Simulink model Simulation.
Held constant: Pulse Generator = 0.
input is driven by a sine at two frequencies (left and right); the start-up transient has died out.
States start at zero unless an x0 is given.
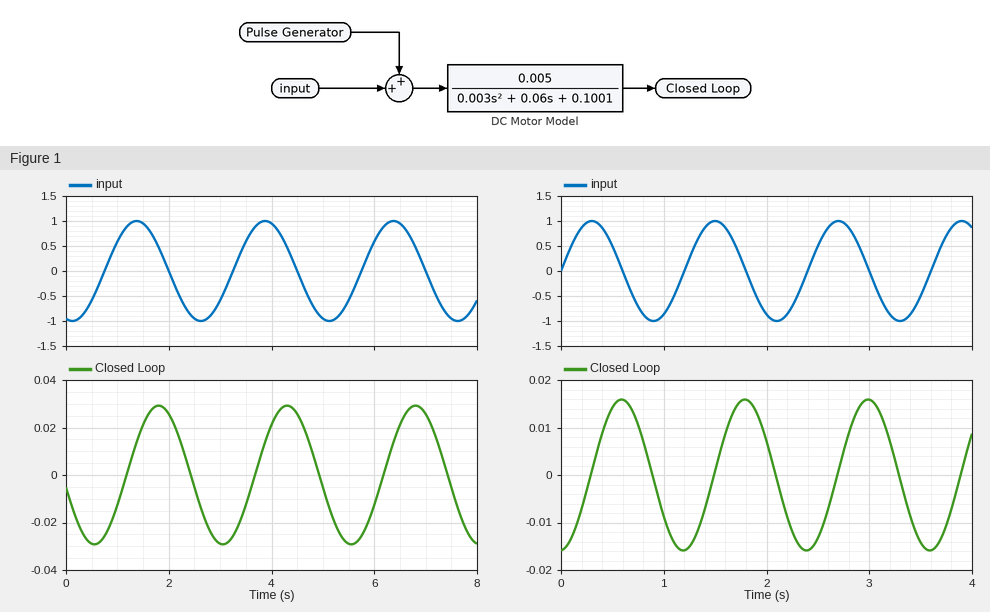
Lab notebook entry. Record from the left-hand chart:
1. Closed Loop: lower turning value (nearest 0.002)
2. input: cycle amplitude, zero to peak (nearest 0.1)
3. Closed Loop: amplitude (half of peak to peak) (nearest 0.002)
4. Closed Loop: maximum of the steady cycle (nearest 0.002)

-0.030
1.0
0.030
0.030
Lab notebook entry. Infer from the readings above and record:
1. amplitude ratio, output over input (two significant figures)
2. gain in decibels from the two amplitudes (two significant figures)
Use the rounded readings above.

0.030
-30 dB
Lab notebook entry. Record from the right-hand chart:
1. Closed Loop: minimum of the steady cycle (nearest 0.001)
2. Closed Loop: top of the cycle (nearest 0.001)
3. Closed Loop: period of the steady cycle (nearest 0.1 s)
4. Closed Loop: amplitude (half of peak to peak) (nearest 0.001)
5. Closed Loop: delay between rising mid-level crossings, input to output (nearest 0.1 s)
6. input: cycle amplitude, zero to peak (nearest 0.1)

-0.016
0.016
1.2 s
0.016
0.3 s
1.0
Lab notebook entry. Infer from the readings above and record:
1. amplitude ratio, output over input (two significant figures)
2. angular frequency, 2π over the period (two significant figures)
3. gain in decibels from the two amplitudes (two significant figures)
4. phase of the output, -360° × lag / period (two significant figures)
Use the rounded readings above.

0.016
5.2 rad/s
-36 dB
-90°
